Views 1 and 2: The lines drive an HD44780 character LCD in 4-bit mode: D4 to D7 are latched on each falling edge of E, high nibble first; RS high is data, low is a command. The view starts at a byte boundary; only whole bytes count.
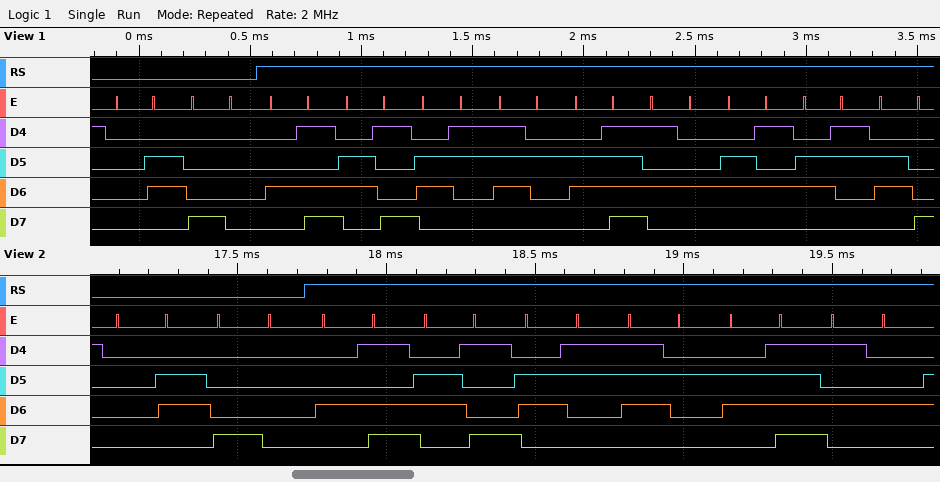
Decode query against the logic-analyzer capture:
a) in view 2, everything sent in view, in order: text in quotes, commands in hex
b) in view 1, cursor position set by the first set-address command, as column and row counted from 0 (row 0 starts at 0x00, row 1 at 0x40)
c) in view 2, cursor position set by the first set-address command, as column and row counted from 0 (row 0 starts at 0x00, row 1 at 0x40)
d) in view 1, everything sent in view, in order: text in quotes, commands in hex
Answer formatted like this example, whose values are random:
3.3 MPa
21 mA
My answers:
0x06 0x80 "MicroT"
column 0, row 0
column 0, row 0
0x06 0x80 "MicroTech"
